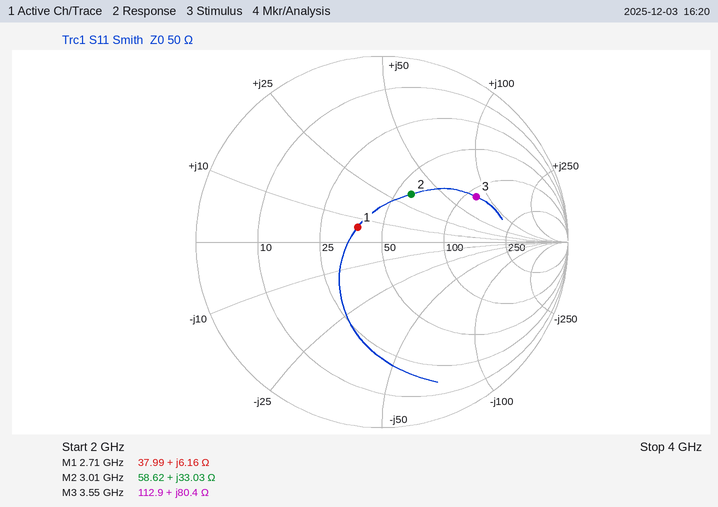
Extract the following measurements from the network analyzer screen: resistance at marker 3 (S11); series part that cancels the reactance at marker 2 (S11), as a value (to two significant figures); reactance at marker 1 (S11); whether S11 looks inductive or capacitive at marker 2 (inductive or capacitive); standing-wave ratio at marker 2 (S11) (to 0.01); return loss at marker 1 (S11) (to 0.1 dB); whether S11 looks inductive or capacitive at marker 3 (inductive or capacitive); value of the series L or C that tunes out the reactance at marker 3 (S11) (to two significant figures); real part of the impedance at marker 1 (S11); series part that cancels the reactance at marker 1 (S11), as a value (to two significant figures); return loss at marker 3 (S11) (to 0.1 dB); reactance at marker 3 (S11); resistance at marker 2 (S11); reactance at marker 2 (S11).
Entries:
112.9 Ω
1.6 pF
+6.16 Ω
inductive
1.86
16.3 dB
inductive
560 fF
37.99 Ω
9.5 pF
5.0 dB
+80.4 Ω
58.62 Ω
+33.03 Ω
